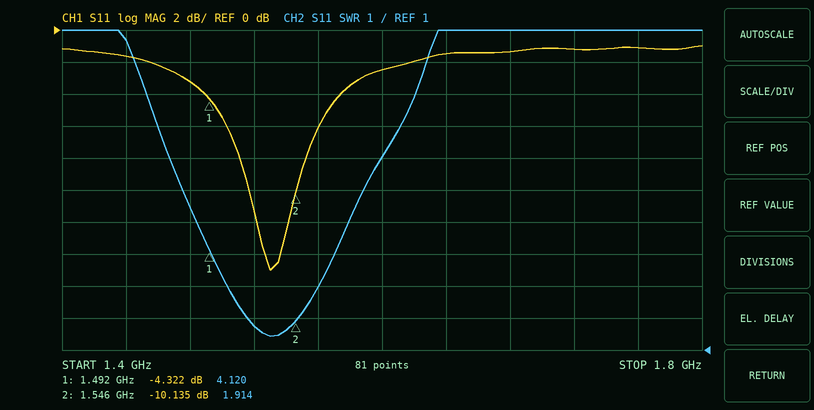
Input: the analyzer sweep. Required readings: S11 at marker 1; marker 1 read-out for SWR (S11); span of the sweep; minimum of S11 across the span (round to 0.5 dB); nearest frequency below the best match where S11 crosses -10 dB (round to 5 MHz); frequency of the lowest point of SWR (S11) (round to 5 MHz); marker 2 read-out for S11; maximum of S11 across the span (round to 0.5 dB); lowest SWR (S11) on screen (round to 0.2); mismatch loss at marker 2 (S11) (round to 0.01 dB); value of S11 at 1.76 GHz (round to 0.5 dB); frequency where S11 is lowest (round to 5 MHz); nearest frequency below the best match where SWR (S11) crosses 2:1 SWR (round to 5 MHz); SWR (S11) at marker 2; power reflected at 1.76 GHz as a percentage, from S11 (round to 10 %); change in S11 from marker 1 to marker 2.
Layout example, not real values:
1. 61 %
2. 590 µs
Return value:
1. -4.322 dB
2. 4.120
3. 400 MHz
4. -15.0 dB
5. 1.515 GHz
6. 1.530 GHz
7. -10.135 dB
8. -1.0 dB
9. 1.4
10. 0.44 dB
11. -1.0 dB
12. 1.530 GHz
13. 1.515 GHz
14. 1.914
15. 80 %
16. -5.813 dB
